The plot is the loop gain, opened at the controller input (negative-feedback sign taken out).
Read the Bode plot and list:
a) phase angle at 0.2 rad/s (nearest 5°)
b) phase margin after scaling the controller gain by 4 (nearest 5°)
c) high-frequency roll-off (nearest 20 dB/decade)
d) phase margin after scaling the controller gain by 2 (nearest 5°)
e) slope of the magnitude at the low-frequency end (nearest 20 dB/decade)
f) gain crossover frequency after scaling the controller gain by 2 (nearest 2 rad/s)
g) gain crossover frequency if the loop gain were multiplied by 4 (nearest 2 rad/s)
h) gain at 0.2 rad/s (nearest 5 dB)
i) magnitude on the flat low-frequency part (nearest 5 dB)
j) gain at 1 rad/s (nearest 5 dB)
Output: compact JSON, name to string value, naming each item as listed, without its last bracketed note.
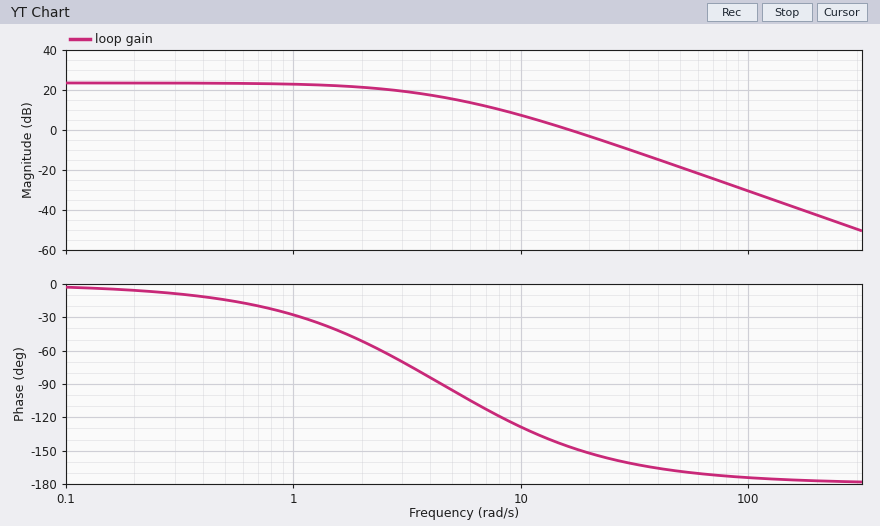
{"phase angle at 0.2 rad/s": "-5°", "phase margin after scaling the controller gain by 4": "15°", "high-frequency roll-off": "-40 dB/decade", "phase margin after scaling the controller gain by 2": "25°", "slope of the magnitude at the low-frequency end": "0 dB/decade", "gain crossover frequency after scaling the controller gain by 2": "24 rad/s", "gain crossover frequency if the loop gain were multiplied by 4": "34 rad/s", "gain at 0.2 rad/s": "25 dB", "magnitude on the flat low-frequency part": "25 dB", "gain at 1 rad/s": "25 dB"}
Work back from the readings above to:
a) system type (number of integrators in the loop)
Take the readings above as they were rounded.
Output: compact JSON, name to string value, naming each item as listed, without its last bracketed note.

{"system type": "0"}
